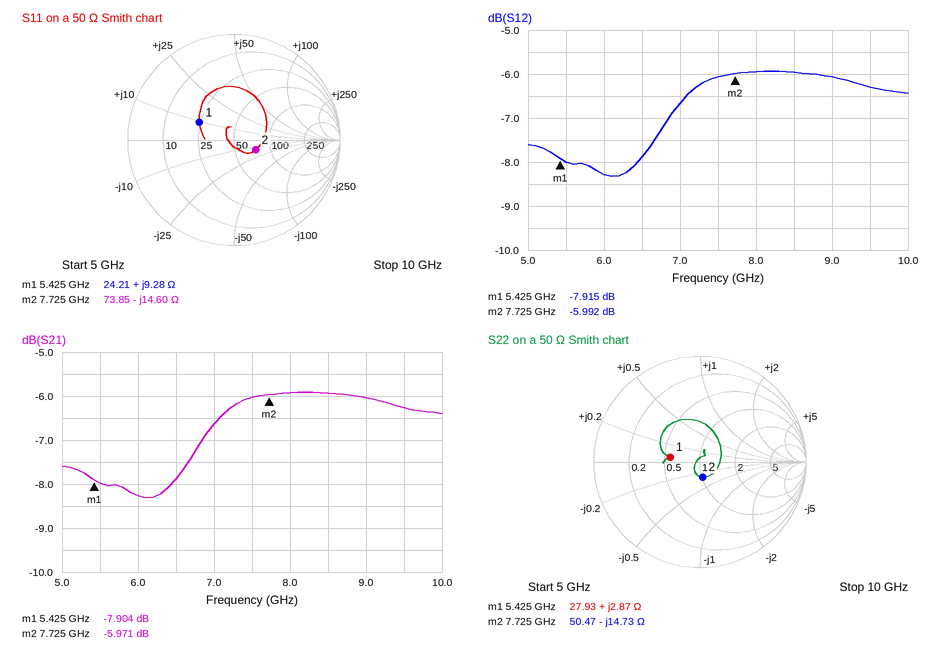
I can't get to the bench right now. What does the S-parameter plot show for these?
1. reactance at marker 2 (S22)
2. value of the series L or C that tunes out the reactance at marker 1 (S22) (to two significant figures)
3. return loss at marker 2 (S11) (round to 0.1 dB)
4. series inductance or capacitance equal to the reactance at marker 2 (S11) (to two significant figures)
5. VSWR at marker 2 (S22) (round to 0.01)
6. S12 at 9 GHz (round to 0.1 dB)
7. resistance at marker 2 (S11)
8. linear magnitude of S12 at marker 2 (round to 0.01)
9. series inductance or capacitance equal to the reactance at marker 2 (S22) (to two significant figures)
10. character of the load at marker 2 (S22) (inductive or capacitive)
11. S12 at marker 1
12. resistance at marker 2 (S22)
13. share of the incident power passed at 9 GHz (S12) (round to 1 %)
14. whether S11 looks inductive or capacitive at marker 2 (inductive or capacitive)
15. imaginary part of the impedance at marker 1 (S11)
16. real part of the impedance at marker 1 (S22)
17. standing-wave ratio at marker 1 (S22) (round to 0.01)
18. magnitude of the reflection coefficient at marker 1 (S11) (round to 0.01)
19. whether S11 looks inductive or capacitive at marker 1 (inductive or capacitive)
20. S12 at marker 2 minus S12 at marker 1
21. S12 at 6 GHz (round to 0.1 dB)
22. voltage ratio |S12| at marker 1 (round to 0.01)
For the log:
-14.73 Ω
10 pF
13.0 dB
1.4 pF
1.34
-6.1 dB
73.85 Ω
0.50
1.4 pF
capacitive
-7.915 dB
50.47 Ω
25 %
capacitive
+9.28 Ω
27.93 Ω
1.80
0.37
inductive
1.923 dB
-8.3 dB
0.40
